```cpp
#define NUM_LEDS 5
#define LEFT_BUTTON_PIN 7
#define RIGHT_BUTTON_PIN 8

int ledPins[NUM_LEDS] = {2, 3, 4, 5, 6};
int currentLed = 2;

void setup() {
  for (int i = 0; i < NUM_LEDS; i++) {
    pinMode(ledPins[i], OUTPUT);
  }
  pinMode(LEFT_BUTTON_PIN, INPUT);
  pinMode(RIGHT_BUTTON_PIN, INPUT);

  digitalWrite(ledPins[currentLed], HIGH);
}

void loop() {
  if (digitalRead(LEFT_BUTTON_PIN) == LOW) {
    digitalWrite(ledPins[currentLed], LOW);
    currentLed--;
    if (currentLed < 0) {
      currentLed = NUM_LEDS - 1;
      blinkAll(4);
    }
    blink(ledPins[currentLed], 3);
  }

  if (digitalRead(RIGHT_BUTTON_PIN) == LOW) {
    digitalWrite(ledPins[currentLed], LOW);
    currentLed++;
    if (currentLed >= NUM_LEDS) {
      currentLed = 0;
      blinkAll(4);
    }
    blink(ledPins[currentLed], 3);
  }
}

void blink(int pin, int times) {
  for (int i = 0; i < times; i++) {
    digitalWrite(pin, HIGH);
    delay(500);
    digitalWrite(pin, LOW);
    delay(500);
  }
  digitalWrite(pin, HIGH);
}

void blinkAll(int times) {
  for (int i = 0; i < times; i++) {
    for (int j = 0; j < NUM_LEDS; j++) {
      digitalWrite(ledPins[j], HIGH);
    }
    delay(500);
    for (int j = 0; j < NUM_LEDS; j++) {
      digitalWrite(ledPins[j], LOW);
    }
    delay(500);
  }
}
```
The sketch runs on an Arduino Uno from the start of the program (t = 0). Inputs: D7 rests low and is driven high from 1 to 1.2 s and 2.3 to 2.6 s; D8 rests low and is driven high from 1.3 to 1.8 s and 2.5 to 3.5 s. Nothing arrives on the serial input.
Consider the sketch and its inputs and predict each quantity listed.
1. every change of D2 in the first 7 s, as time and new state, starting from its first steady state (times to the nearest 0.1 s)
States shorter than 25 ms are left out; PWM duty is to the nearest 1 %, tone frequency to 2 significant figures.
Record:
0 s low; 3 s high; 3.5 s low; 4 s high; 4.5 s low; 5 s high; 5.5 s low
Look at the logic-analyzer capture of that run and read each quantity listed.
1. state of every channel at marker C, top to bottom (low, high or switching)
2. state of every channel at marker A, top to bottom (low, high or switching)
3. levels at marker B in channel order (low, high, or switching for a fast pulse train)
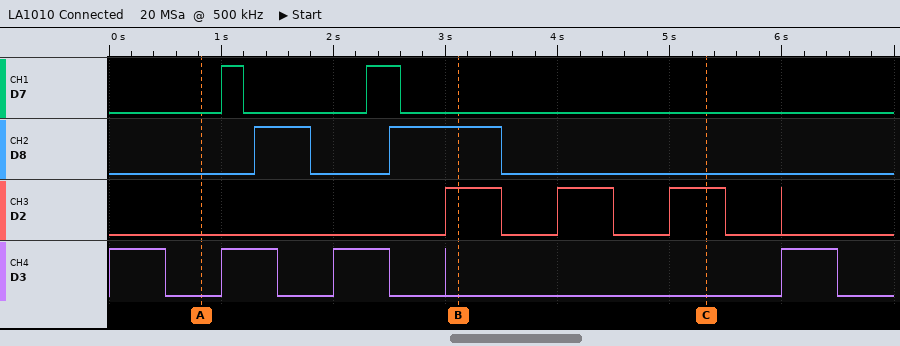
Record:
D7 low, D8 low, D2 high, D3 low
D7 low, D8 low, D2 low, D3 low
D7 low, D8 high, D2 high, D3 low
